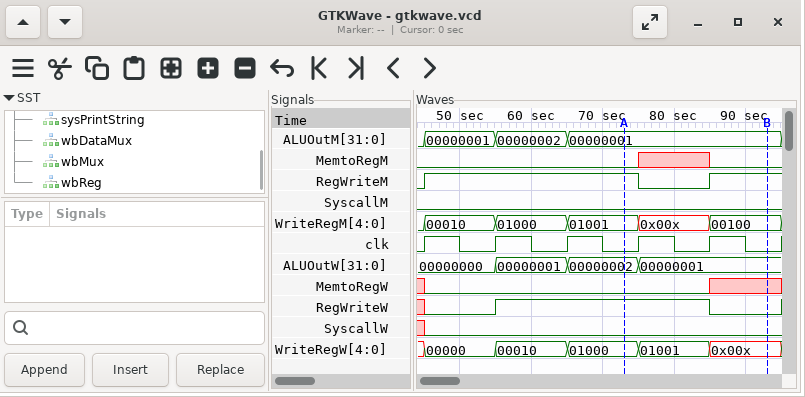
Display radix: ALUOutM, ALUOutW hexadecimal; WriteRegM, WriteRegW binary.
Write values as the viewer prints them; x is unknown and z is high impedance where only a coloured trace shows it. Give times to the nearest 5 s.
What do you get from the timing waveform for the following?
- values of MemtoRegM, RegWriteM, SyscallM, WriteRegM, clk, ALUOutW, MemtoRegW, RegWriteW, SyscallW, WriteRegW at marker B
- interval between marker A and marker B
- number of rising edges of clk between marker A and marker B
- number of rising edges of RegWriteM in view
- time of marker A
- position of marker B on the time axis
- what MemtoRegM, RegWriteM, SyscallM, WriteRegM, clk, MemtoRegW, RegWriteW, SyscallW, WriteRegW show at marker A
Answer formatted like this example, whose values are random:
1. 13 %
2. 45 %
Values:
1. MemtoRegM=0, RegWriteM=1, SyscallM=0, WriteRegM=00100, clk=0, ALUOutW=00000001, MemtoRegW=x, RegWriteW=0, SyscallW=0, WriteRegW=0x00x
2. 20 s
3. 2
4. 2
5. 75 s
6. 95 s
7. MemtoRegM=0, RegWriteM=1, SyscallM=0, WriteRegM=01001, clk=0, MemtoRegW=0, RegWriteW=1, SyscallW=0, WriteRegW=01000
